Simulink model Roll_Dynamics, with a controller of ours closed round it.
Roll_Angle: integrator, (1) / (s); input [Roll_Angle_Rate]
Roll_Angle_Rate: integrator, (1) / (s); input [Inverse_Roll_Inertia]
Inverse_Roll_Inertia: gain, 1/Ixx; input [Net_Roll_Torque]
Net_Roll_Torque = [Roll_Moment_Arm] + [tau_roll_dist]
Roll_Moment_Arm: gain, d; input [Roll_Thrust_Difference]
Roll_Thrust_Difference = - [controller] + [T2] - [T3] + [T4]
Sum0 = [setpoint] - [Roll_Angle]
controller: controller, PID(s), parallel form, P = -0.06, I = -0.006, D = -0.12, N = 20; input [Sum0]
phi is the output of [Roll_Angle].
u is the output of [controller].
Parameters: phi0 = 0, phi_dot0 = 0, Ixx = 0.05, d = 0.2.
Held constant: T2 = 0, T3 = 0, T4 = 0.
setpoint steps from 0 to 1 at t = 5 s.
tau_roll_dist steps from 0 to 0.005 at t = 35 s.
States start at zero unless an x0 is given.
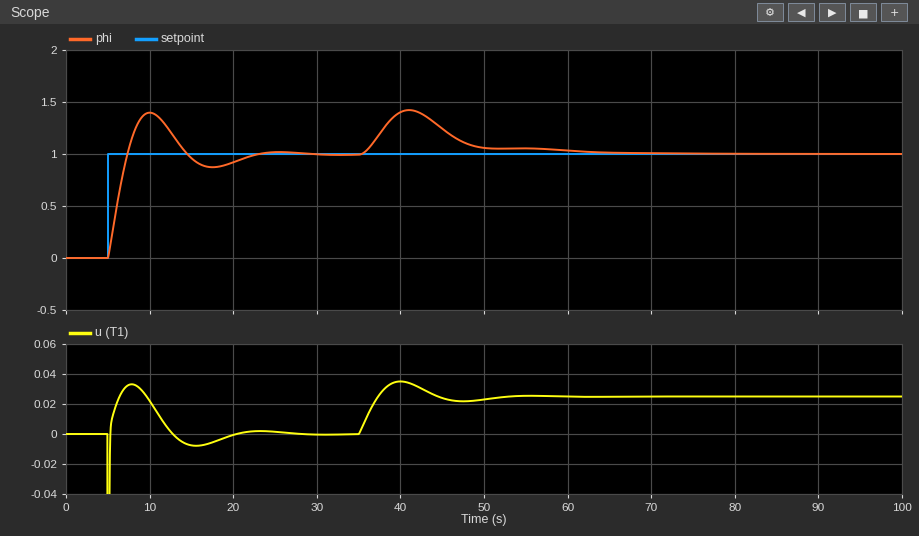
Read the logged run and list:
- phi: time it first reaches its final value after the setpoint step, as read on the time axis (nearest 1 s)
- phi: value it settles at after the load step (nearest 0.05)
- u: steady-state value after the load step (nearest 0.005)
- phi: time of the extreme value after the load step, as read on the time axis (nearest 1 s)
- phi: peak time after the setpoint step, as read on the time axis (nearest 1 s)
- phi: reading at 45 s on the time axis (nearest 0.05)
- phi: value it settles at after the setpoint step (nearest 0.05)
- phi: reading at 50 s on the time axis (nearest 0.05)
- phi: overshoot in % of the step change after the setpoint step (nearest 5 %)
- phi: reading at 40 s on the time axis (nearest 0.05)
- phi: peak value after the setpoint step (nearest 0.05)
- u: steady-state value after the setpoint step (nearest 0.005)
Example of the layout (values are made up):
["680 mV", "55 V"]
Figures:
["7 s", "1.00", "0.025", "41 s", "10 s", "1.25", "1.00", "1.05", "40 %", "1.40", "1.40", "0.000"]
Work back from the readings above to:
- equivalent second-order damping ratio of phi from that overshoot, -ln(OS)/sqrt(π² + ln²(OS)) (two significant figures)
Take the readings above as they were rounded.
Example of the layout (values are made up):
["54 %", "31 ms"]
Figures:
["0.28"]
